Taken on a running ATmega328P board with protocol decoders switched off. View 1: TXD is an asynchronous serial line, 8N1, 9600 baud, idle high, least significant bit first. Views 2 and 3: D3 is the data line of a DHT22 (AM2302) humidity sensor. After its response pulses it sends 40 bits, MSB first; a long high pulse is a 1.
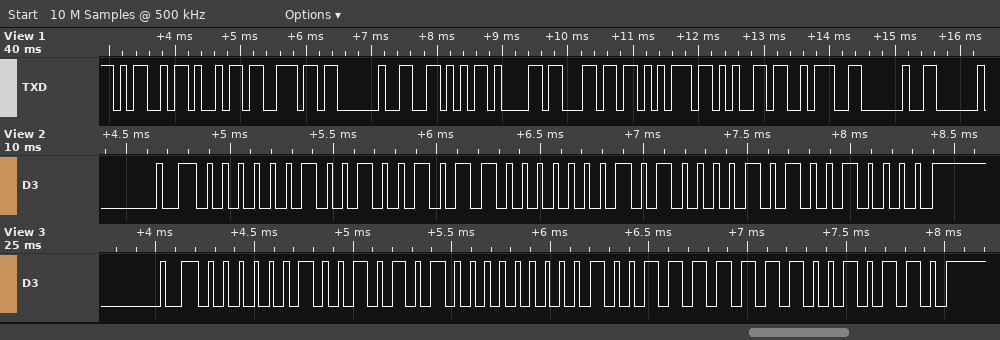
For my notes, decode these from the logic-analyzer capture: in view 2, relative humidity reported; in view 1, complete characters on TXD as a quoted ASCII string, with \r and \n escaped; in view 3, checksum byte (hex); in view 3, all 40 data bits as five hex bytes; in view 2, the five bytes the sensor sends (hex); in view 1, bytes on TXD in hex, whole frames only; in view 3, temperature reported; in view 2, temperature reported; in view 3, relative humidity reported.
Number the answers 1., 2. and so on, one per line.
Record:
1. 58.7 %
2. "Min Value: "
3. 0x96
4. 02 54 01 3F 96
5. 02 4B 01 42 90
6. 0x4D 0x69 0x6E 0x20 0x56 0x61 0x6C 0x75 0x65 0x3A 0x20
7. 31.9 °C
8. 32.2 °C
9. 59.6 %
